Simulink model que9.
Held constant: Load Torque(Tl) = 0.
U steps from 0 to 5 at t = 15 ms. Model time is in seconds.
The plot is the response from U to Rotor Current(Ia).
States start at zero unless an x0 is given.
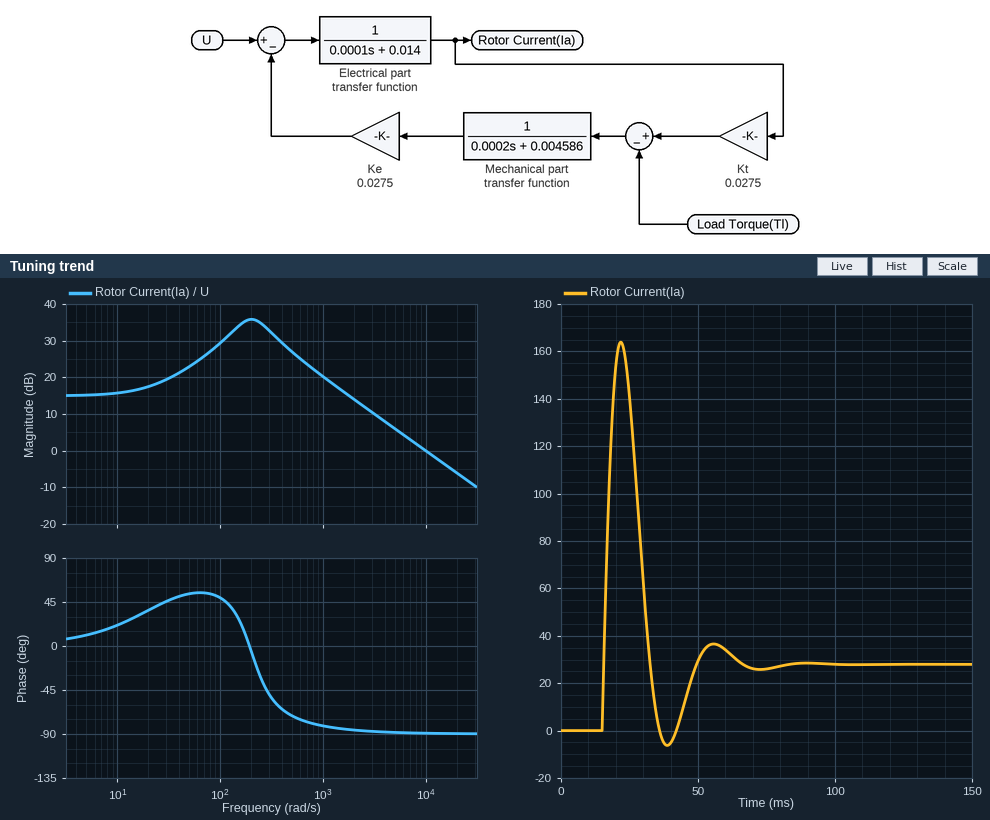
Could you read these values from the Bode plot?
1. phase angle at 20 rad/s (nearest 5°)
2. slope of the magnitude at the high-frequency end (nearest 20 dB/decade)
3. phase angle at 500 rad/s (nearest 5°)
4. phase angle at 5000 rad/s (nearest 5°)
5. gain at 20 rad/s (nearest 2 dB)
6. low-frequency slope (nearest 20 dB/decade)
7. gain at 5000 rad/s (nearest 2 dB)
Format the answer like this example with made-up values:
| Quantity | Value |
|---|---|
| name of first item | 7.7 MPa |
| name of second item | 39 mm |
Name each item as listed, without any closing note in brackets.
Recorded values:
| Quantity | Value |
|---|---|
| phase angle at 20 rad/s | 35° |
| slope of the magnitude at the high-frequency end | -20 dB/decade |
| phase angle at 500 rad/s | -70° |
| phase angle at 5000 rad/s | -90° |
| gain at 20 rad/s | 18 dB |
| low-frequency slope | 0 dB/decade |
| gain at 5000 rad/s | 6 dB |
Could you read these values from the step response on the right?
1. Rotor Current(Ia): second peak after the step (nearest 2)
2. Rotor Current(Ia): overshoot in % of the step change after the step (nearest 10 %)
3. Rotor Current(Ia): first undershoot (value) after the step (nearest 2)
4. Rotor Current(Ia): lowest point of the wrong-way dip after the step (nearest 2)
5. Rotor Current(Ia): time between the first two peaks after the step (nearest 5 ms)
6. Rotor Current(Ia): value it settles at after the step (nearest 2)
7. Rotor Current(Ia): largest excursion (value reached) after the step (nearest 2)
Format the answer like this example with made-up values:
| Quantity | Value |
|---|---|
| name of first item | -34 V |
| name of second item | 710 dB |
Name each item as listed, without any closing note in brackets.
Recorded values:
| Quantity | Value |
|---|---|
| Rotor Current(Ia): second peak after the step | 36 |
| Rotor Current(Ia): overshoot in % of the step change after the step | 490 % |
| Rotor Current(Ia): first undershoot (value) after the step | -6 |
| Rotor Current(Ia): lowest point of the wrong-way dip after the step | -6 |
| Rotor Current(Ia): time between the first two peaks after the step | 35 ms |
| Rotor Current(Ia): value it settles at after the step | 28 |
| Rotor Current(Ia): largest excursion (value reached) after the step | 164 |
